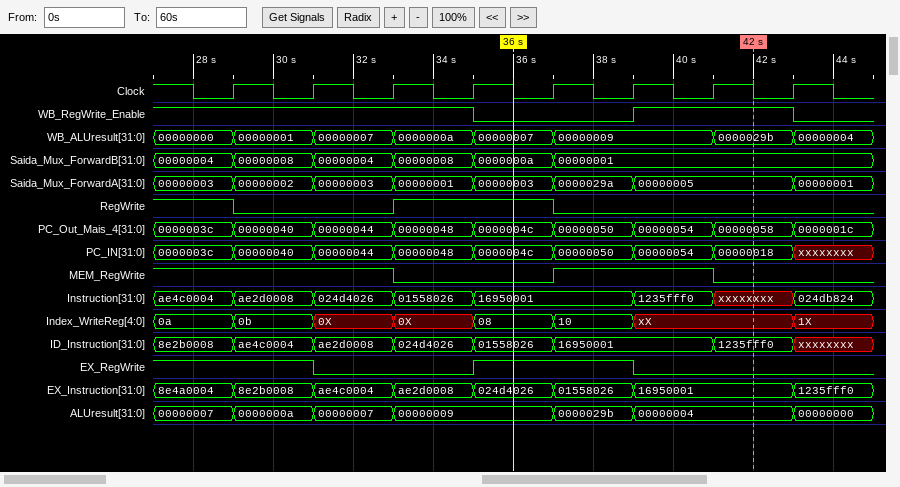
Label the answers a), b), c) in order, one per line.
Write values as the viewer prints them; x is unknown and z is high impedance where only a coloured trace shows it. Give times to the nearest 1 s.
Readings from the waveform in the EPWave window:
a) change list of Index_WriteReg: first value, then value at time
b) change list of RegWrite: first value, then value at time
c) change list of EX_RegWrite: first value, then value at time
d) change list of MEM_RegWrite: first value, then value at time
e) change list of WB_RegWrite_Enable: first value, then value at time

a) 0a, 0b at 29 s, 0X at 31 s, 0X at 33 s, 08 at 35 s, 10 at 37 s, xX at 39 s, 1X at 43 s
b) 1, 0 at 29 s, 1 at 33 s, 0 at 37 s
c) 1, 0 at 31 s, 1 at 35 s, 0 at 39 s
d) 1, 0 at 33 s, 1 at 37 s, 0 at 41 s
e) 1, 0 at 35 s, 1 at 39 s, 0 at 43 s
